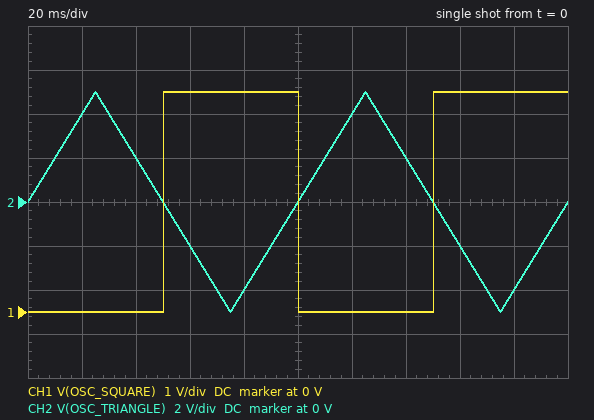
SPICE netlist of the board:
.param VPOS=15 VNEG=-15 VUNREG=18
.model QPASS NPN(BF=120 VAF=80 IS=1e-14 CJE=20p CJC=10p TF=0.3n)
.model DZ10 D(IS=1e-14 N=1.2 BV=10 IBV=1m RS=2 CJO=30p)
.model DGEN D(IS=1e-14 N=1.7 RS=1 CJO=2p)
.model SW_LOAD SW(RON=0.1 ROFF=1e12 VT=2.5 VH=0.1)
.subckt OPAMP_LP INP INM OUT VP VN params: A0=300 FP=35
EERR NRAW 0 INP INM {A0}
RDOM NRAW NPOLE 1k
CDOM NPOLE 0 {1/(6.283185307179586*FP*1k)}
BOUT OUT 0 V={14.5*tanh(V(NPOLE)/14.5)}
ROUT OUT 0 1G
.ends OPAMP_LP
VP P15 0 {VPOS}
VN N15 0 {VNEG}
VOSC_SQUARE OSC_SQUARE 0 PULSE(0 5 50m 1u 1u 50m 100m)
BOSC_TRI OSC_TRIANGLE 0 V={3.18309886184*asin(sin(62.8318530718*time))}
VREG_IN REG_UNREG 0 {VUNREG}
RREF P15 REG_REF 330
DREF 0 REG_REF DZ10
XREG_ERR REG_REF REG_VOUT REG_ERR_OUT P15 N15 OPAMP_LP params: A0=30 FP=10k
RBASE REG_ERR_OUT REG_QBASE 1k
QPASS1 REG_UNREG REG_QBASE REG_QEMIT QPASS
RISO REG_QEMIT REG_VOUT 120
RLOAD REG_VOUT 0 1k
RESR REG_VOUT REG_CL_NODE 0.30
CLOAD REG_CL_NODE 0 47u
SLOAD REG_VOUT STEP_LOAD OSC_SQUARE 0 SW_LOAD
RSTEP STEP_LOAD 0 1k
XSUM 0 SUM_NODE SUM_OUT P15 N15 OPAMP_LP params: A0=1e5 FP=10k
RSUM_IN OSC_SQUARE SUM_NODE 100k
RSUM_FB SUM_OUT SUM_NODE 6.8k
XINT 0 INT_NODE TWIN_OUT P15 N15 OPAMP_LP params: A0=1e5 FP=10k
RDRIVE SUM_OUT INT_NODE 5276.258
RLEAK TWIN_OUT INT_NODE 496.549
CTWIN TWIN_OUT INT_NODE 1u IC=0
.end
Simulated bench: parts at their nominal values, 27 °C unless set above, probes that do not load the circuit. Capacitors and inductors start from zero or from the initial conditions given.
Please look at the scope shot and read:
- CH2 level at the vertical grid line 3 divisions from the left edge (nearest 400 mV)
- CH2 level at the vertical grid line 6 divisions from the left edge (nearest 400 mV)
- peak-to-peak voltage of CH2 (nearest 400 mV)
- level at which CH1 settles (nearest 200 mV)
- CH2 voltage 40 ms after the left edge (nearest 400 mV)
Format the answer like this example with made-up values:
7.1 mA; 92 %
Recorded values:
-2.0 V; 4.0 V; 10.0 V; 5.0 V; 2.0 V
